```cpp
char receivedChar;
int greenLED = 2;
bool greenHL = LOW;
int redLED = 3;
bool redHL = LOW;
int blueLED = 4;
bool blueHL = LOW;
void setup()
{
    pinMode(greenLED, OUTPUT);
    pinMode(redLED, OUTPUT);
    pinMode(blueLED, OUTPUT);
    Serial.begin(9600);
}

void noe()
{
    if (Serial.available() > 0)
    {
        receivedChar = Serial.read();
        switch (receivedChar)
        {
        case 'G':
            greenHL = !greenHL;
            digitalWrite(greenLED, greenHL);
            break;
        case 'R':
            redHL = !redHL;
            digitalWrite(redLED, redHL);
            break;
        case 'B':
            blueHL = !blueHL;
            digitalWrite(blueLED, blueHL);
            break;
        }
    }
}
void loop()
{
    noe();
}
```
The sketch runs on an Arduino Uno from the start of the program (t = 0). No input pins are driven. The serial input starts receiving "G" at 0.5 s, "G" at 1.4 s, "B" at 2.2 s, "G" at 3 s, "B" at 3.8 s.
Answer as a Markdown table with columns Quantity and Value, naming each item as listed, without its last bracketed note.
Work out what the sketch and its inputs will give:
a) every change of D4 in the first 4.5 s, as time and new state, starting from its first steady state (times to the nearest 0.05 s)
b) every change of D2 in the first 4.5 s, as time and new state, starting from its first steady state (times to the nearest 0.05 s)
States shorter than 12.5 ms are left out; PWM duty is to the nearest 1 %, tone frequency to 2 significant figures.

| Quantity | Value |
|---|---|
| every change of D4 in the first 4.5 s, as time and new state, starting from its first steady state | 0 s low; 2.2 s high; 3.8 s low |
| every change of D2 in the first 4.5 s, as time and new state, starting from its first steady state | 0 s low; 0.5 s high; 1.4 s low; 3 s high |
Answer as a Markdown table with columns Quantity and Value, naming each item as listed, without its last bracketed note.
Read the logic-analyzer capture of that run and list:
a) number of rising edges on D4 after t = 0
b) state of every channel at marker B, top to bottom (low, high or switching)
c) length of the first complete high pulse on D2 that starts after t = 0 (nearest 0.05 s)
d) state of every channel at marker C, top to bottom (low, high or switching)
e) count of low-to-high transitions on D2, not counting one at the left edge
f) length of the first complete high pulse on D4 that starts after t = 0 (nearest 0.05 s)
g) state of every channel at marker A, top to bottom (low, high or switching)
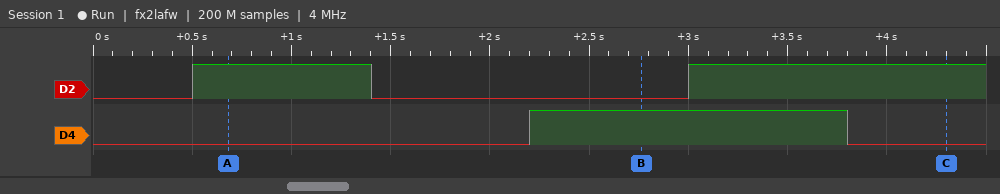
| Quantity | Value |
|---|---|
| number of rising edges on D4 after t = 0 | 1 |
| state of every channel at marker B, top to bottom | D2 low, D4 high |
| length of the first complete high pulse on D2 that starts after t = 0 | 0.90 s |
| state of every channel at marker C, top to bottom | D2 high, D4 low |
| count of low-to-high transitions on D2, not counting one at the left edge | 2 |
| length of the first complete high pulse on D4 that starts after t = 0 | 1.60 s |
| state of every channel at marker A, top to bottom | D2 high, D4 low |
